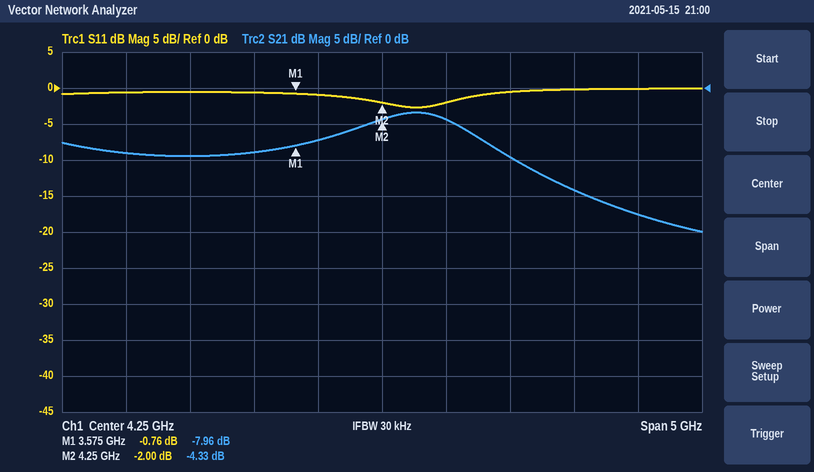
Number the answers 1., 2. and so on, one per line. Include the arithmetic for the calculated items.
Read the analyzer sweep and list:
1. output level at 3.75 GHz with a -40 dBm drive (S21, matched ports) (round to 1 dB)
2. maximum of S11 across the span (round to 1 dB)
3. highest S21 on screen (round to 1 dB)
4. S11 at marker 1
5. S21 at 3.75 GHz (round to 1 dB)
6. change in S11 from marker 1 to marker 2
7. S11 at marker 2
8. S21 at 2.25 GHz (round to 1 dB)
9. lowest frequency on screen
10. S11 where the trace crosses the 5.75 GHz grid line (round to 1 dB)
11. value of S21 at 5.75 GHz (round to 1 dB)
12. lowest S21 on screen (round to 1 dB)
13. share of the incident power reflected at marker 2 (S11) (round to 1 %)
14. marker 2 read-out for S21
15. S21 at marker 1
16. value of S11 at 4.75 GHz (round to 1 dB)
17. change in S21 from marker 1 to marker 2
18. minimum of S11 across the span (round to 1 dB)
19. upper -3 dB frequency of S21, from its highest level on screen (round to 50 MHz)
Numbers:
1. -40 dBm + (-7 dB) = -47 dBm
2. 0 dB
3. -3 dB
4. -0.76 dB
5. -7 dB
6. -2 − (-0.76) = -1.24 dB
7. -2.00 dB
8. -9 dB
9. 1.75 GHz
10. 0 dB
11. -14 dB
12. -20 dB
13. 10^(-2/10) ≈ 63 %
14. -4.33 dB
15. -7.96 dB
16. -2 dB
17. -4.33 − (-7.96) = 3.63 dB
18. -3 dB
19. 4.95 GHz
